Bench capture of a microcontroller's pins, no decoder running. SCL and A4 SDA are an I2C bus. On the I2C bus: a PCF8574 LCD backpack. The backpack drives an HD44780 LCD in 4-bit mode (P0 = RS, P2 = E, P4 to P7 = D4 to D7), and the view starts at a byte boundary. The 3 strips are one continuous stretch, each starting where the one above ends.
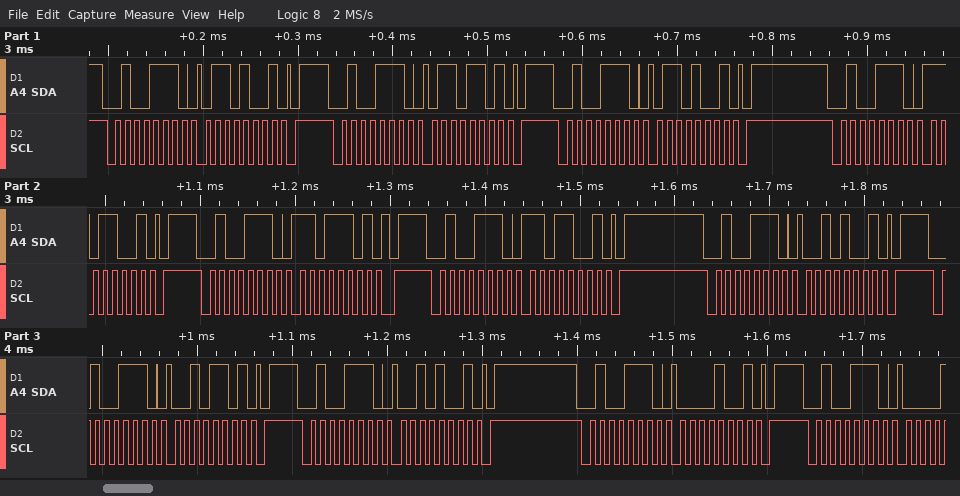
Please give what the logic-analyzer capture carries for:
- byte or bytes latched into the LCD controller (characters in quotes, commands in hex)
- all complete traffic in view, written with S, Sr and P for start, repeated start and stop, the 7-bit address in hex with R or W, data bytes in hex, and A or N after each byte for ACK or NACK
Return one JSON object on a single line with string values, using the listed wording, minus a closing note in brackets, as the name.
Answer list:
{"byte or bytes latched into the LCD controller": "'m'", "all complete traffic in view, written with S, Sr and P for start, repeated start and stop, the 7-bit address in hex with R or W, data bytes in hex, and A or N after each byte for ACK or NACK": "S 27W A 69 A P S 27W A 6D A P S 27W A 69 A P S 27W A D9 A P S 27W A DD A P S 27W A D9 A P S 27W A 29 A P S 27W A 2D A P S 27W A 29 A P S 27W A 09 A P S 27W A"}
